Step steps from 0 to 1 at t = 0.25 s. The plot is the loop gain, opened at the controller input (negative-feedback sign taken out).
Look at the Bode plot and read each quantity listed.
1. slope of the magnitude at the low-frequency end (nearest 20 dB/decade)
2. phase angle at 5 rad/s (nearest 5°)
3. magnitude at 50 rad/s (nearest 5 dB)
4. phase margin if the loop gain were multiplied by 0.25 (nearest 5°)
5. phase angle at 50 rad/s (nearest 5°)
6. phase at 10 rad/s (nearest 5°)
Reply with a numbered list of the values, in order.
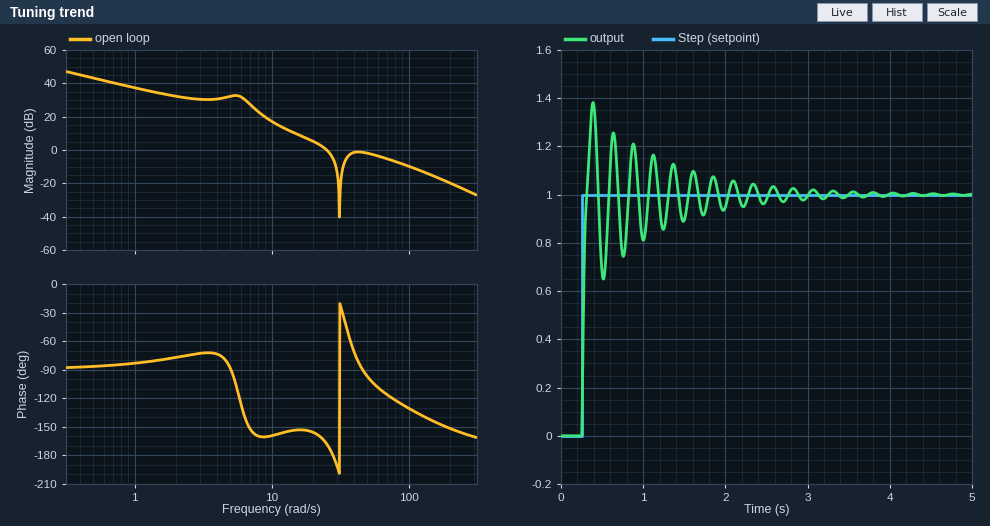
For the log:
1. -20 dB/decade
2. -90°
3. 0 dB
4. 25°
5. -95°
6. -160°
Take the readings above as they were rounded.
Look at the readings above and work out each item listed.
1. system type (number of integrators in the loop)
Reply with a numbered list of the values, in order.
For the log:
1. 1
